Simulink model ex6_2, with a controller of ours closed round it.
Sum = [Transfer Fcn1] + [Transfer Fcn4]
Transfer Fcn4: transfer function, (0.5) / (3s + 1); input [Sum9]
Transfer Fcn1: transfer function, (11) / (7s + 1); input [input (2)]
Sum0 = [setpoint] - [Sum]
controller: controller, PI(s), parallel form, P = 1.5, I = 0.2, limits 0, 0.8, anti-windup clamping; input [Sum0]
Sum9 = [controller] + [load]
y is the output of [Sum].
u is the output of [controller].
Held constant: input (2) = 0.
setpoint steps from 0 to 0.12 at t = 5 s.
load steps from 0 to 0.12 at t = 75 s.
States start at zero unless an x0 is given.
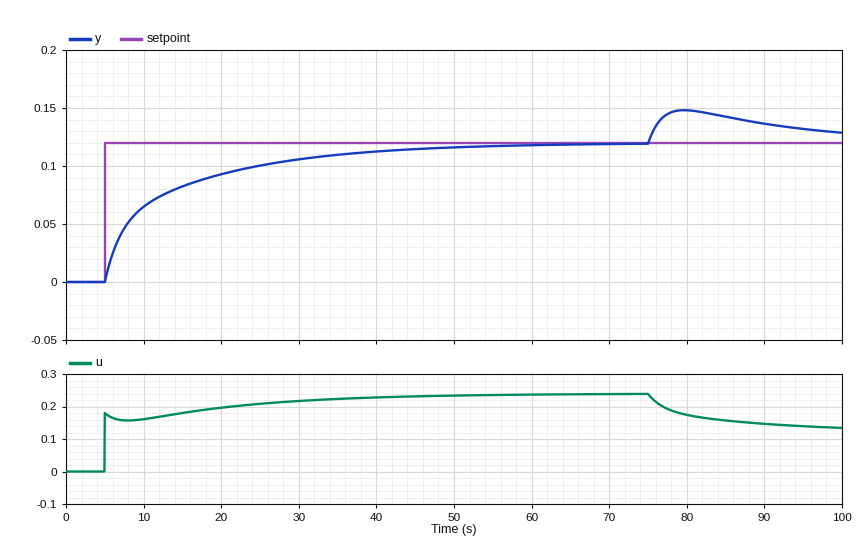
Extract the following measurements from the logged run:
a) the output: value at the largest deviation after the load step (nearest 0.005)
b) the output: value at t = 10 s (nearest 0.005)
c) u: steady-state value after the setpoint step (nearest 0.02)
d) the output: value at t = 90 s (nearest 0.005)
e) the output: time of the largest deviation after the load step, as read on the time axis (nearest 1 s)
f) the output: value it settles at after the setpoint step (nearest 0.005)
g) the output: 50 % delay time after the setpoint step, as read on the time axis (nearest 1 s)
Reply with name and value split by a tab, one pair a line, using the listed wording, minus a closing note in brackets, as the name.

the output: value at the largest deviation after the load step	0.150
the output: value at t = 10 s	0.065
u: steady-state value after the setpoint step	0.24
the output: value at t = 90 s	0.135
the output: time of the largest deviation after the load step, as read on the time axis	80 s
the output: value it settles at after the setpoint step	0.120
the output: 50 % delay time after the setpoint step, as read on the time axis	9 s
